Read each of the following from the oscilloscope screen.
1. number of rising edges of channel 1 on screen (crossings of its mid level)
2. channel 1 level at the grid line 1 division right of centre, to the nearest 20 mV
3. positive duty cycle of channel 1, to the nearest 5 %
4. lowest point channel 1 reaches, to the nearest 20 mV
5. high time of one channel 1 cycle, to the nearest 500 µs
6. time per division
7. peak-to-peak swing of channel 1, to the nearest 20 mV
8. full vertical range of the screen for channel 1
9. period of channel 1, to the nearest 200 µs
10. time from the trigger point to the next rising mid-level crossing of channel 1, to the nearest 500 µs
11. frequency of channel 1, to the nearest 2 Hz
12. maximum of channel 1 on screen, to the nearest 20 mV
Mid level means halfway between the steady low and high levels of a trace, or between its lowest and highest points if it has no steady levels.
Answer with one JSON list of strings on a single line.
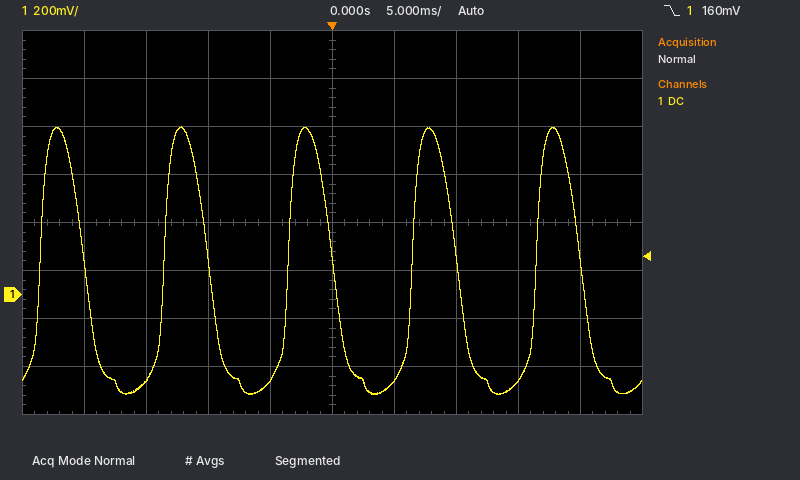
["5", "-360 mV", "35 %", "-420 mV", "3.5 ms", "5 ms", "1.12 V", "1.6 V", "10.0 ms", "6.5 ms", "100 Hz", "700 mV"]
